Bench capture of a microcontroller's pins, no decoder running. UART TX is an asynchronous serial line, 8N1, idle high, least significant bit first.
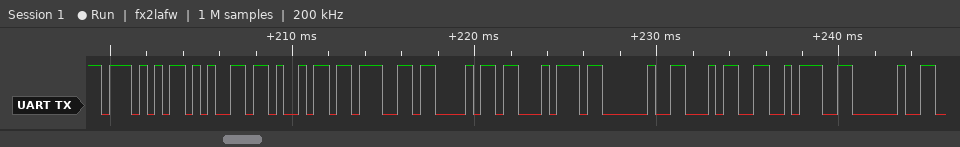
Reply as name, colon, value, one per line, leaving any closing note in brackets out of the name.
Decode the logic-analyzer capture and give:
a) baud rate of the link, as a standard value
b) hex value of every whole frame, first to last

baud rate of the link, as a standard value: 2400 baud
hex value of every whole frame, first to last: 0x57 0x65 0x69 0x67 0x68 0x74 0x20 0x34 0x3A 0x20
